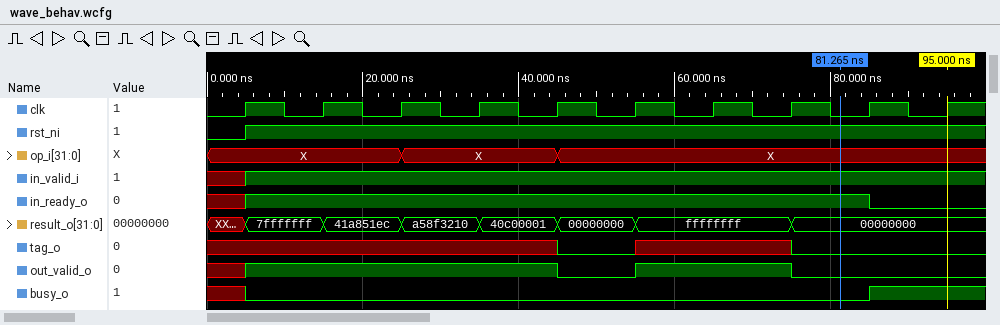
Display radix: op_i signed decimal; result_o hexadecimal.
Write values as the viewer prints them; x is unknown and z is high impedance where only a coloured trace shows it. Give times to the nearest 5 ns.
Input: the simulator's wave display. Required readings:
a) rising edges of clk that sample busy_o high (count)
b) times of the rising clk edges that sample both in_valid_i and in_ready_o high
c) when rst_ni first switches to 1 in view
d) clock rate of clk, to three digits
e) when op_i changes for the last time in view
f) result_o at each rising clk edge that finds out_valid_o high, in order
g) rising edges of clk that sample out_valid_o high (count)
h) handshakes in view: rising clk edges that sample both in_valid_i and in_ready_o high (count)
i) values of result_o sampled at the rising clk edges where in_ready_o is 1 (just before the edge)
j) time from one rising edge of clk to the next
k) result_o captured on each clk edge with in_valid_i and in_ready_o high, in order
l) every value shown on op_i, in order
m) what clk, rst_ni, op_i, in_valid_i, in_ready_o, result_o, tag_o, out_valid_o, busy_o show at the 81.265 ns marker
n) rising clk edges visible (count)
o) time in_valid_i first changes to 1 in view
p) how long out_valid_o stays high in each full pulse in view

1
15 ns, 25 ns, 35 ns, 45 ns, 55 ns, 65 ns, 75 ns, 85 ns
5 ns
100 MHz
45 ns
7fffffff, 41a851ec, a58f3210, 40c00001, ffffffff, ffffffff
6
8
7fffffff, 41a851ec, a58f3210, 40c00001, 00000000, ffffffff, ffffffff, 00000000
10 ns
7fffffff, 41a851ec, a58f3210, 40c00001, 00000000, ffffffff, ffffffff, 00000000
X, X, X
clk=0, rst_ni=1, op_i=X, in_valid_i=1, in_ready_o=1, result_o=00000000, tag_o=0, out_valid_o=0, busy_o=0
10
5 ns
20 ns
